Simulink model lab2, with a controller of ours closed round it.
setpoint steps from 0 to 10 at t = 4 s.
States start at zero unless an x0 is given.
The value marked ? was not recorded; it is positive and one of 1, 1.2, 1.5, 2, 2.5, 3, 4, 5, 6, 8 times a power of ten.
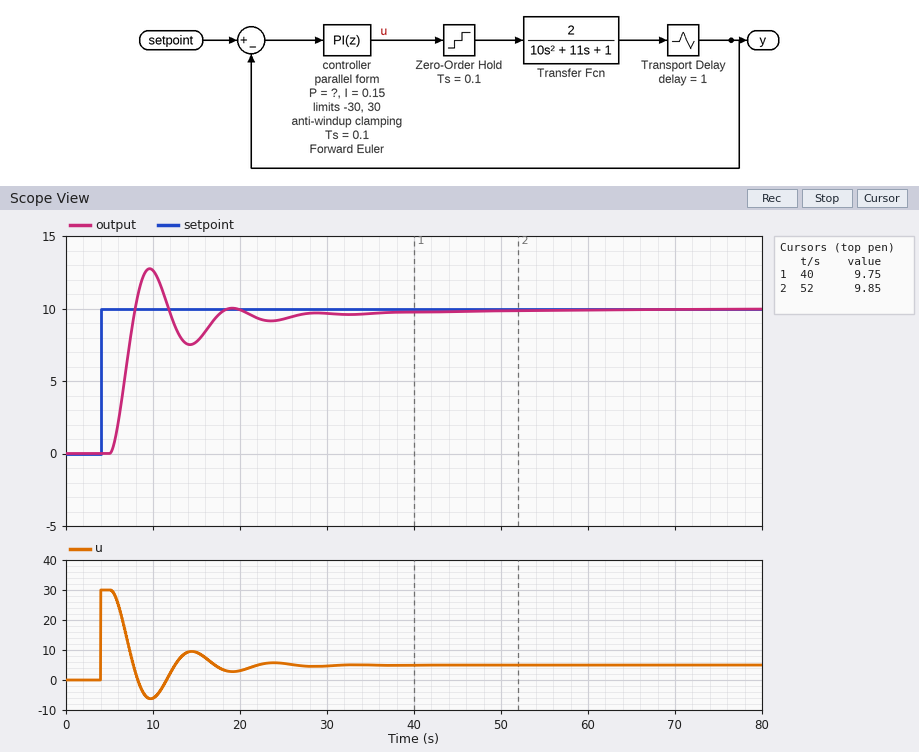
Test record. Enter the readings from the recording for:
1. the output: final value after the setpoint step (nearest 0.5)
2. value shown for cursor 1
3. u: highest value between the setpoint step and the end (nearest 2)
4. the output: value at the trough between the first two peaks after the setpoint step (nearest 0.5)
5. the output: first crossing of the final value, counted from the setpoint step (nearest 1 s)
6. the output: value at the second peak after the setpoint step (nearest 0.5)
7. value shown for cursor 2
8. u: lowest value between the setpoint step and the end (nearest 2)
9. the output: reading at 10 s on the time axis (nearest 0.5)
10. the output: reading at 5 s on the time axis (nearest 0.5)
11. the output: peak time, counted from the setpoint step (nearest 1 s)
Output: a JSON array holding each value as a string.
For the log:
["10.0", "9.75", "30", "7.5", "4 s", "10.0", "9.85", "-6", "12.5", "0.0", "6 s"]
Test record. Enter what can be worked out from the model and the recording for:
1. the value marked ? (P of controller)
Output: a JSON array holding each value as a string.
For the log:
["3"]
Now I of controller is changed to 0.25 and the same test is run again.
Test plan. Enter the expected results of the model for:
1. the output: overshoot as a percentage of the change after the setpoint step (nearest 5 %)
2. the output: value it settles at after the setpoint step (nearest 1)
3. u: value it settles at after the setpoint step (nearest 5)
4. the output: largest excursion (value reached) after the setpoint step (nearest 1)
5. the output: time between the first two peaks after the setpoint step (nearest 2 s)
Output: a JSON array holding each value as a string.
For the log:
["30 %", "10", "5", "13", "10 s"]
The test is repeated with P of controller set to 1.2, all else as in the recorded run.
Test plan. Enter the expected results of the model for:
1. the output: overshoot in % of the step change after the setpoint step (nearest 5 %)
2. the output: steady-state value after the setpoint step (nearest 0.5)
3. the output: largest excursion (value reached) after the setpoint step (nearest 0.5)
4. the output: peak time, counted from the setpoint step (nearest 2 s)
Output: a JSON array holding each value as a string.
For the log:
["10 %", "10.0", "11.0", "10 s"]
